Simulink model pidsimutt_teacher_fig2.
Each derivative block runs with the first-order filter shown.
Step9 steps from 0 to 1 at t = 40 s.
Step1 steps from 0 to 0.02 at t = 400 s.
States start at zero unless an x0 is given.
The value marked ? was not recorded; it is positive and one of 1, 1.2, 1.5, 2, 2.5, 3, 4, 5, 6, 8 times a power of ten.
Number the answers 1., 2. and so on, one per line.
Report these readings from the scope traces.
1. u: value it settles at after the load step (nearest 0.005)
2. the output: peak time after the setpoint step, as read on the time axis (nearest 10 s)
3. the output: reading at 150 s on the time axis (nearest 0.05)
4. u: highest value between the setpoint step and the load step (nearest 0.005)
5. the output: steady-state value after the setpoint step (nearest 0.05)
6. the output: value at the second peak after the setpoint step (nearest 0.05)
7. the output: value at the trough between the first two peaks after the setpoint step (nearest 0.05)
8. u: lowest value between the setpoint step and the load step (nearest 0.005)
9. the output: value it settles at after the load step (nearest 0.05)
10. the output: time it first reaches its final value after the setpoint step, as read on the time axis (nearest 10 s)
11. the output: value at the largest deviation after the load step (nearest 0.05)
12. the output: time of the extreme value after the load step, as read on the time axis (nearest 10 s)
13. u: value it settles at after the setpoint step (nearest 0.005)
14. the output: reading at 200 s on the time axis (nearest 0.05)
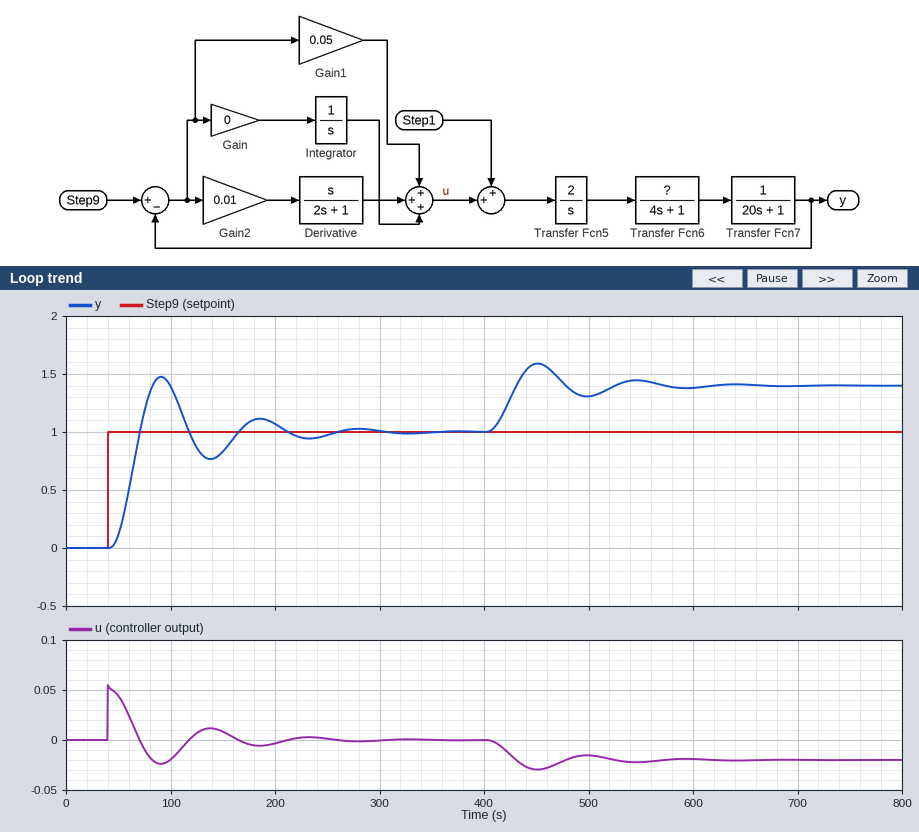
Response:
1. -0.020
2. 90 s
3. 0.85
4. 0.055
5. 1.00
6. 1.10
7. 0.75
8. -0.025
9. 1.40
10. 70 s
11. 1.60
12. 450 s
13. 0.000
14. 1.05
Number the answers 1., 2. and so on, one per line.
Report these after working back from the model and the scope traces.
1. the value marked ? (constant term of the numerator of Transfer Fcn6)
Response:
1. 1
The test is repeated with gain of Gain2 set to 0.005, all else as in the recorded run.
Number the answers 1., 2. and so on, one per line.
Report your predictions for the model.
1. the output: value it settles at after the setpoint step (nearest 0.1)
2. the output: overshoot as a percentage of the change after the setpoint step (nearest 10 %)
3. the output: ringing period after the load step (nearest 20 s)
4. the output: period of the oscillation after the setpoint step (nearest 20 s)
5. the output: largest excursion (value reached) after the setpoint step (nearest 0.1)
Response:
1. 1.0
2. 50 %
3. 100 s
4. 100 s
5. 1.5
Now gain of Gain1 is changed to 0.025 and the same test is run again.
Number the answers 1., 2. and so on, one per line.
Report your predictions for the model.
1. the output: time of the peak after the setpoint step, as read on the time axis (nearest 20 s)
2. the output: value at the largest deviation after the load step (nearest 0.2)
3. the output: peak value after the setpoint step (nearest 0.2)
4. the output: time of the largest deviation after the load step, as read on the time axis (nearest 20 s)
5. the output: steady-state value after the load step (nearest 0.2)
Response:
1. 120 s
2. 2.0
3. 1.2
4. 480 s
5. 1.8
